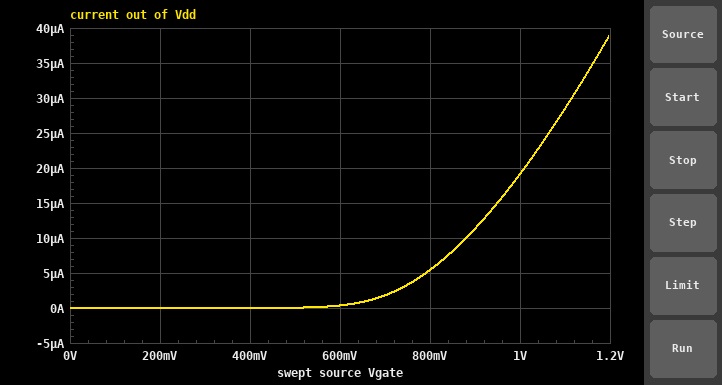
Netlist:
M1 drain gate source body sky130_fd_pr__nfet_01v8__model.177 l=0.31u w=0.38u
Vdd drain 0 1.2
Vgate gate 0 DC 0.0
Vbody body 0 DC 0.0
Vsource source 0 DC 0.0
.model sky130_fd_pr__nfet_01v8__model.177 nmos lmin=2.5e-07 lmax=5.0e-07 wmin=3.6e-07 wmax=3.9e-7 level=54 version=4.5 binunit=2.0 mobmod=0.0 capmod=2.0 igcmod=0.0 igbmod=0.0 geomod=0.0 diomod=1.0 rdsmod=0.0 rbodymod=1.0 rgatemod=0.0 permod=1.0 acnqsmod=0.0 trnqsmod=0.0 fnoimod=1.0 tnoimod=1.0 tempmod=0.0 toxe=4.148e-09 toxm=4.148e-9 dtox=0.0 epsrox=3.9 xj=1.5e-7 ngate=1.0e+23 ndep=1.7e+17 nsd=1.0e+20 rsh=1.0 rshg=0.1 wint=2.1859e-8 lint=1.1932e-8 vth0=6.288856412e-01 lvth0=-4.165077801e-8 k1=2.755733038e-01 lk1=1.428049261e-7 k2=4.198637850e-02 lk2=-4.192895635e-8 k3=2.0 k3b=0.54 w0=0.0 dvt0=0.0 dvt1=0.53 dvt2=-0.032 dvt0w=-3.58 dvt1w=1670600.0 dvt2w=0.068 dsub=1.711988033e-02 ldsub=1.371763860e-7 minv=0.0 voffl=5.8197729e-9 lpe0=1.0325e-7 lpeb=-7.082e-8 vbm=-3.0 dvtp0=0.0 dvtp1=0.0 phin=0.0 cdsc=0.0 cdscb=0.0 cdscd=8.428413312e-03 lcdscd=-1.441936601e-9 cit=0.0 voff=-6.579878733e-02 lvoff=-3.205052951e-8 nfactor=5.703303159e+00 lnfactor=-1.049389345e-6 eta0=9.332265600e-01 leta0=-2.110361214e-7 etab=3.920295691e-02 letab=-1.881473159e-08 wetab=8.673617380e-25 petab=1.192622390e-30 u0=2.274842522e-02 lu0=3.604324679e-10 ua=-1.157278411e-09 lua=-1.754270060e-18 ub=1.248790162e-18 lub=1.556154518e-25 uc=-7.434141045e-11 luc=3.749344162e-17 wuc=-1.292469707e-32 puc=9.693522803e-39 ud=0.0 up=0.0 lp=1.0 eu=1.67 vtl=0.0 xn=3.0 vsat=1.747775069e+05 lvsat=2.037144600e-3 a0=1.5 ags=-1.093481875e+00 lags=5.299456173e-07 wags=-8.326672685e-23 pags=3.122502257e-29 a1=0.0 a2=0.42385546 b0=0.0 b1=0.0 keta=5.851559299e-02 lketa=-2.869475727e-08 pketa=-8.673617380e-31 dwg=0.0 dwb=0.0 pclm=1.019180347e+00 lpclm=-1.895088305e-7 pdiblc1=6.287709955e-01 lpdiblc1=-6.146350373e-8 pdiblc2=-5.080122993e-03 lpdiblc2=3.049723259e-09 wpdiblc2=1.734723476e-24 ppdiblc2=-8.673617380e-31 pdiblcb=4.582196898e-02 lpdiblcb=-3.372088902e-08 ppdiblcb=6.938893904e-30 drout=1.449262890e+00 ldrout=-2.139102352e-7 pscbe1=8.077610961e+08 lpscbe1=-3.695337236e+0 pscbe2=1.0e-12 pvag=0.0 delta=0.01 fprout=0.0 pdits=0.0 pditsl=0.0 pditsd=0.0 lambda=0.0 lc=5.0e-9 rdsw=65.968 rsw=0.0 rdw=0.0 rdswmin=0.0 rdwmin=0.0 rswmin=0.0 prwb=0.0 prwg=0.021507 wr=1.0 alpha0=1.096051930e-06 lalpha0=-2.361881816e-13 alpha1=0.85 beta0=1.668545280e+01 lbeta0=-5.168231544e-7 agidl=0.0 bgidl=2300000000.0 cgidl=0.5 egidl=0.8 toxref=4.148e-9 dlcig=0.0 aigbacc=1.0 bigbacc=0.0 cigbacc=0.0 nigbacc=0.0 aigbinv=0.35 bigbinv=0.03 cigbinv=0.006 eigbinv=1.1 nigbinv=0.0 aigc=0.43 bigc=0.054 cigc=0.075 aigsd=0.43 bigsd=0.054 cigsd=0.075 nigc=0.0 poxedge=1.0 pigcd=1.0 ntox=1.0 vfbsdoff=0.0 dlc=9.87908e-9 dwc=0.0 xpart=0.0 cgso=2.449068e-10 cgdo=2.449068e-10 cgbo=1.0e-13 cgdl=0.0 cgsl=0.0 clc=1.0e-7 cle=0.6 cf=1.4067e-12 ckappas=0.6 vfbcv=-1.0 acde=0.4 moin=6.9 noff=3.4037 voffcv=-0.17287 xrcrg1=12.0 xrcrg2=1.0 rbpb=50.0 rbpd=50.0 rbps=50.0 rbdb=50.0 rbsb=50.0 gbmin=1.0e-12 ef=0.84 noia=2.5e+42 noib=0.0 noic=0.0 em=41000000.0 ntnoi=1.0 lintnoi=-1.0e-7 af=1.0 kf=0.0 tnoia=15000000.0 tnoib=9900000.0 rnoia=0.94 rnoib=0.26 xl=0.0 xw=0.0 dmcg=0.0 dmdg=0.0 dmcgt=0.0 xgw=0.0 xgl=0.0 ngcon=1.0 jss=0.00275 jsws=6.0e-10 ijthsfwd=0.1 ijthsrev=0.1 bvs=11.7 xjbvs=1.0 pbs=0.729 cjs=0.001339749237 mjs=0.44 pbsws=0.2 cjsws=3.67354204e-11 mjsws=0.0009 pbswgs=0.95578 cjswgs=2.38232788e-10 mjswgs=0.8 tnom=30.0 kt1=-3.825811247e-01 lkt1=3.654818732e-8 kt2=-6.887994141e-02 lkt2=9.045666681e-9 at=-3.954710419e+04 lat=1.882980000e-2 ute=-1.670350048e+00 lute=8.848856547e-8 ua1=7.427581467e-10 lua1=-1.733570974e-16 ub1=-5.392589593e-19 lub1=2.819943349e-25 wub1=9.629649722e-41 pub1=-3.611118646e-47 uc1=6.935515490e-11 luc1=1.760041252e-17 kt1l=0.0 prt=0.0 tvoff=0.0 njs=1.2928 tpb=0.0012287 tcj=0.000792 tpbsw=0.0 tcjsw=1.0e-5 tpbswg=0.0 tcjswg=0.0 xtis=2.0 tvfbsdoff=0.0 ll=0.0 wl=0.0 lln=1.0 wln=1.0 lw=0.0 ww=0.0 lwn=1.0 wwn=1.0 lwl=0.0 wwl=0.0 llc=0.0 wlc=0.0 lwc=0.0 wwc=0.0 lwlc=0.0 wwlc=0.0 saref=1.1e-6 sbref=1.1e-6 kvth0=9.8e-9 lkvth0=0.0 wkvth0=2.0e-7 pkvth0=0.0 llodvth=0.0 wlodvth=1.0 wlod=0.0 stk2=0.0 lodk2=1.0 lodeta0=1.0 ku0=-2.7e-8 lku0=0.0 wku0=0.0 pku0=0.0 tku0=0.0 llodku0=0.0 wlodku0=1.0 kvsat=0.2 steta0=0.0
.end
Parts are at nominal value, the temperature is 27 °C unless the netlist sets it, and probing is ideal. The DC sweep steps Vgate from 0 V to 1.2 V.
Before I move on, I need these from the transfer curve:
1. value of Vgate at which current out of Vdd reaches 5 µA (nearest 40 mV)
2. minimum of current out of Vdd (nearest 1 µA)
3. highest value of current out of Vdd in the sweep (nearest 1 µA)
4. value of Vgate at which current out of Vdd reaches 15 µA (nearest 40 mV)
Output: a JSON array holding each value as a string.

["800 mV", "0 A", "39 µA", "960 mV"]
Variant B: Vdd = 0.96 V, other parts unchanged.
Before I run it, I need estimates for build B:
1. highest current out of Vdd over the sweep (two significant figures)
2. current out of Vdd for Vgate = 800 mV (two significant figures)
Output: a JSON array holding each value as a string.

["38 µA", "5.3 µA"]
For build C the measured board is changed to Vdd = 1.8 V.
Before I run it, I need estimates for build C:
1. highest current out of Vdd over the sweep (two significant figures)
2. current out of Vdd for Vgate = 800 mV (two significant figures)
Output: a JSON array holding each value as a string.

["41 µA", "5.8 µA"]
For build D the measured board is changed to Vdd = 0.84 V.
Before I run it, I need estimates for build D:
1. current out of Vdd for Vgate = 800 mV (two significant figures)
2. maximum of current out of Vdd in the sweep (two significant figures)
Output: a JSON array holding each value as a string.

["5.2 µA", "38 µA"]
